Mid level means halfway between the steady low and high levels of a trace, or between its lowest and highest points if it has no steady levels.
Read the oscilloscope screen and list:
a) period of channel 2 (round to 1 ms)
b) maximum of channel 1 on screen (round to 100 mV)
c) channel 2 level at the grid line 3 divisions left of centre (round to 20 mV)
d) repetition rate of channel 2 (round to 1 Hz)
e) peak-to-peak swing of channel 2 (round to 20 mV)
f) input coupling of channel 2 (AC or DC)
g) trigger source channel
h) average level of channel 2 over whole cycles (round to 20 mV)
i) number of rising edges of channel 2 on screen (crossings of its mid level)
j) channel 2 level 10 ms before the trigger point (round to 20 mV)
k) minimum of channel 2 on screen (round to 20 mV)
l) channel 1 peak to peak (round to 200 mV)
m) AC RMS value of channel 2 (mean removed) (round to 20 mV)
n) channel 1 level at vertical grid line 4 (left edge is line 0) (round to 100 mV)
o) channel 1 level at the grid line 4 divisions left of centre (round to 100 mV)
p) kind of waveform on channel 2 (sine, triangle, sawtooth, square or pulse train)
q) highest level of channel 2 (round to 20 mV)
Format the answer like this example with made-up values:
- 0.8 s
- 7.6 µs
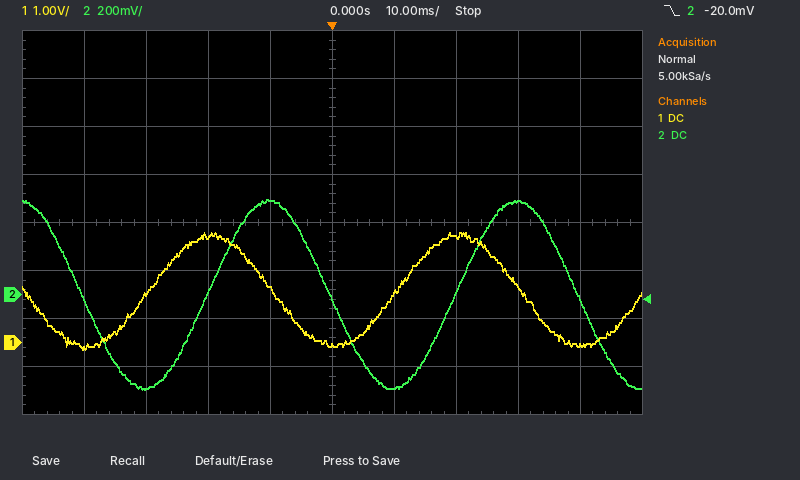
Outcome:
- 40 ms
- 2.3 V
- -400 mV
- 25 Hz
- 800 mV
- DC
- channel 2
- 0 mV
- 2
- 400 mV
- -400 mV
- 2.4 V
- 280 mV
- 1.1 V
- -100 mV
- sine
- 400 mV
